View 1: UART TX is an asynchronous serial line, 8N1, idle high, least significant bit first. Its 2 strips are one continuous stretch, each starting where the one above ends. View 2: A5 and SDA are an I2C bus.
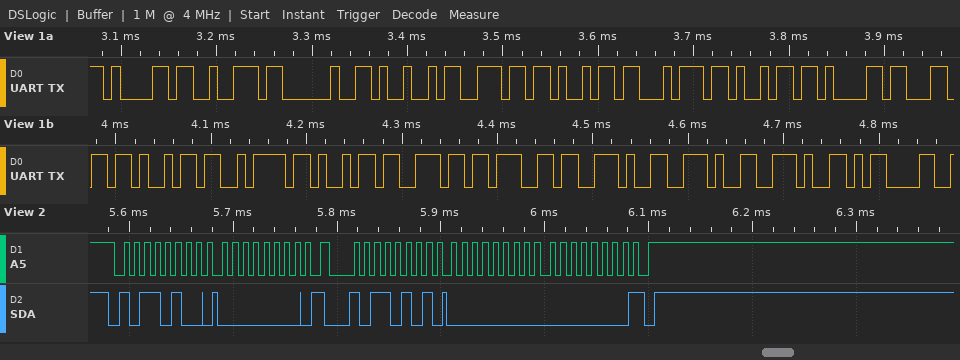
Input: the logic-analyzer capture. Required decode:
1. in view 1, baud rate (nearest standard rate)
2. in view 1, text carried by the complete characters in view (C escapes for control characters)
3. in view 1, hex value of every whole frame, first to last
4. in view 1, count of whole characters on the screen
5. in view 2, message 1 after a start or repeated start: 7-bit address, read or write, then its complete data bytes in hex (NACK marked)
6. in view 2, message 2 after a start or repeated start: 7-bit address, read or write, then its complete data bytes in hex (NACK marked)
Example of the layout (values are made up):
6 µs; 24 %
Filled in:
115200 baud; "ar Initializing...\r"; 61 72 20 49 6E 69 74 69 61 6C 69 7A 69 6E 67 2E 2E 2E 0D; 19; 0x5A write: 00; 0x5A read: 00 00 NACK
